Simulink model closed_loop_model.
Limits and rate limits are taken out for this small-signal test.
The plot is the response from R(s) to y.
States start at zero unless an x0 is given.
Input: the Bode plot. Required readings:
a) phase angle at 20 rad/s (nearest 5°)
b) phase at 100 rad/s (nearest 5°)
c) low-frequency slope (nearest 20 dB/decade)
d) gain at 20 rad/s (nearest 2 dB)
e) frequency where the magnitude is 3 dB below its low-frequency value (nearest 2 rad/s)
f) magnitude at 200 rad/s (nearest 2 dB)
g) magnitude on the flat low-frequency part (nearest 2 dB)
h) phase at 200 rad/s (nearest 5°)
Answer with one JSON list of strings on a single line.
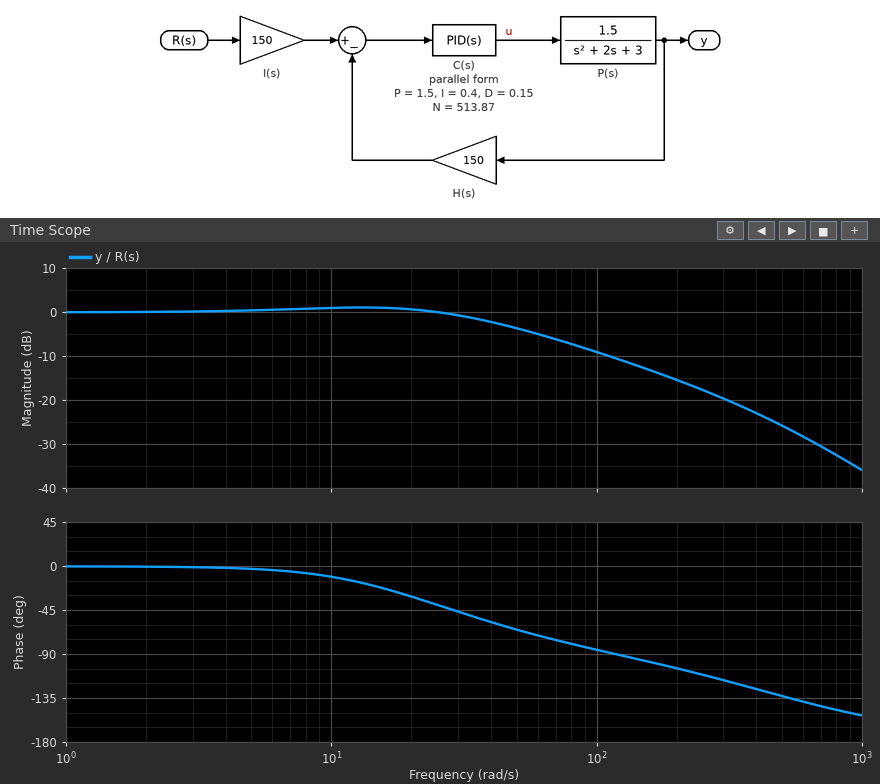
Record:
["-30°", "-85°", "0 dB/decade", "0 dB", "46 rad/s", "-16 dB", "0 dB", "-105°"]
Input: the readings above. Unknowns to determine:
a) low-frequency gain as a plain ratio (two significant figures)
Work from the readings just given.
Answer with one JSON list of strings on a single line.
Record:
["1.0"]
